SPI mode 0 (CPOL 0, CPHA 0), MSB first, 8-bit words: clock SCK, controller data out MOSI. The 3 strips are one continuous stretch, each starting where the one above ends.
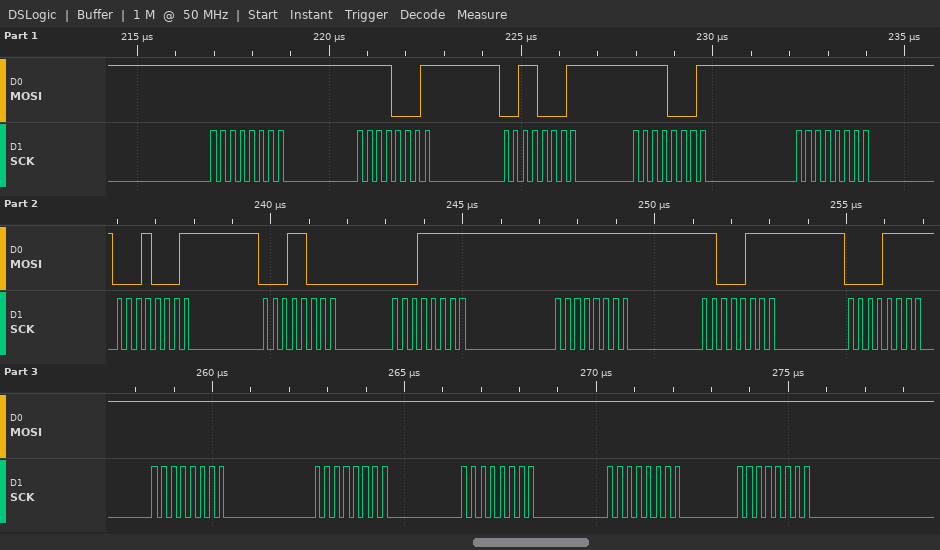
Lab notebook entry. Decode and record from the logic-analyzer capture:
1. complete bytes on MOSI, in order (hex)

FF F1 31 F1 FF 11 18 1F FF C7 0F FF FF FF FF FF
